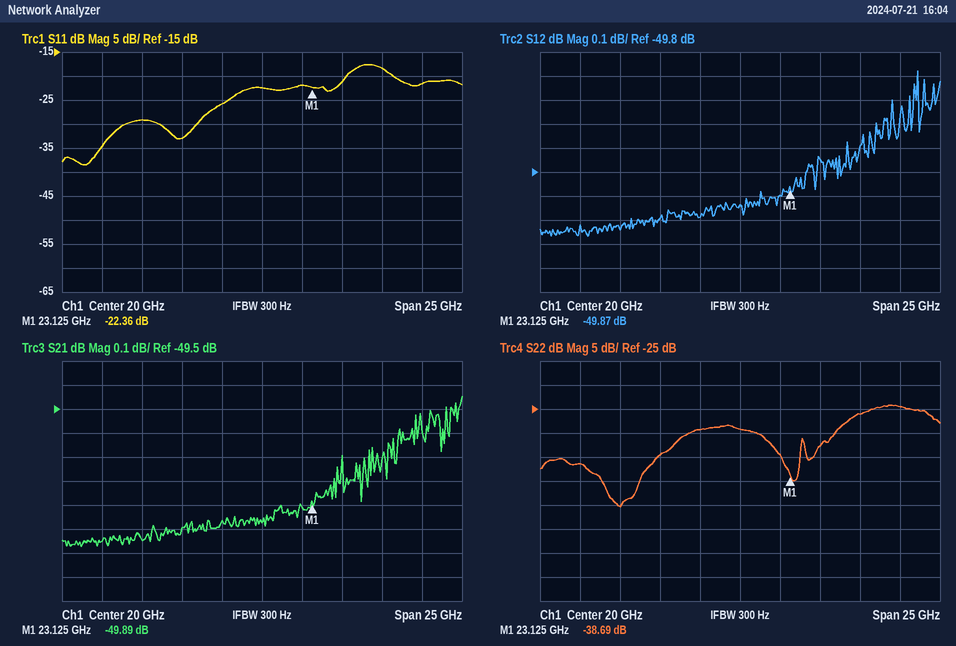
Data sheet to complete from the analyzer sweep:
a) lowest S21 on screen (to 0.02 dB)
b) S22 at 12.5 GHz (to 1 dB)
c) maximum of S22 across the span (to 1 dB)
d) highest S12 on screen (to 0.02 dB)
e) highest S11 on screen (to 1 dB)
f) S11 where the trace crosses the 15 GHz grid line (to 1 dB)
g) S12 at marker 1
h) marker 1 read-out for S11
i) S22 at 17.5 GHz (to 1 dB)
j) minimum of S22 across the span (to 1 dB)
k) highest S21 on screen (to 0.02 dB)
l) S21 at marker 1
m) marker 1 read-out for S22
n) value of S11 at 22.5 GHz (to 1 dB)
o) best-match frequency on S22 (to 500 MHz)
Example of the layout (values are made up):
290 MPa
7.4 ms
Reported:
-50.08 dB
-45 dB
-24 dB
-49.38 dB
-18 dB
-33 dB
-49.87 dB
-22.36 dB
-29 dB
-45 dB
-49.44 dB
-49.89 dB
-38.69 dB
-22 dB
12.5 GHz
